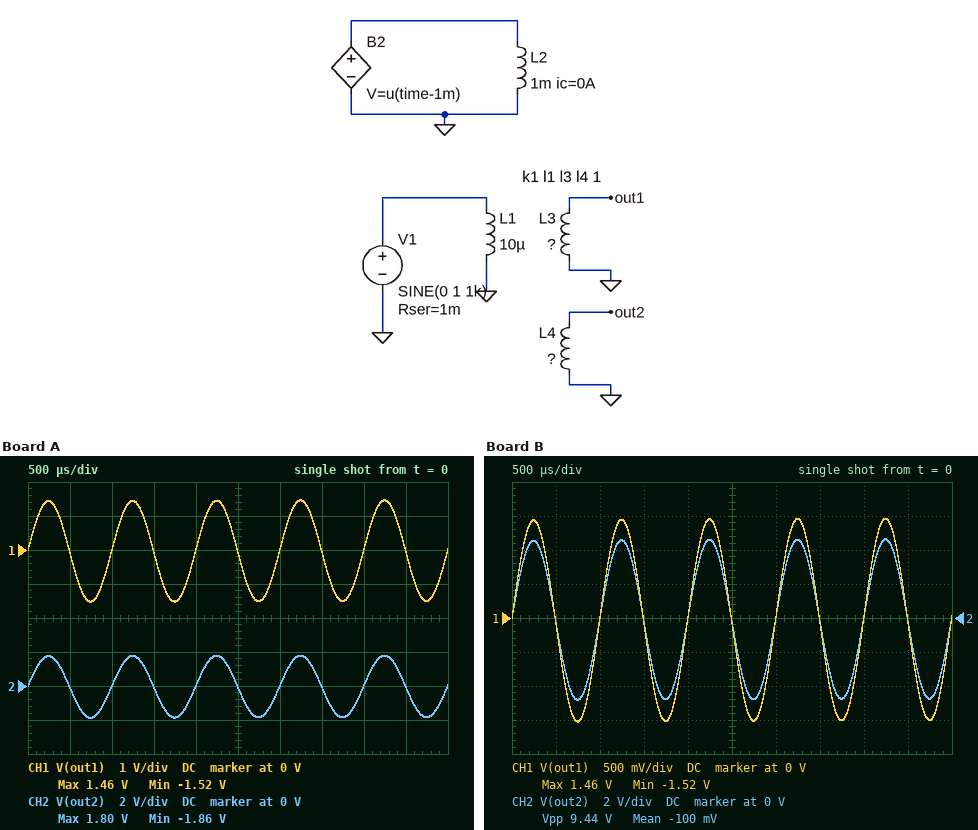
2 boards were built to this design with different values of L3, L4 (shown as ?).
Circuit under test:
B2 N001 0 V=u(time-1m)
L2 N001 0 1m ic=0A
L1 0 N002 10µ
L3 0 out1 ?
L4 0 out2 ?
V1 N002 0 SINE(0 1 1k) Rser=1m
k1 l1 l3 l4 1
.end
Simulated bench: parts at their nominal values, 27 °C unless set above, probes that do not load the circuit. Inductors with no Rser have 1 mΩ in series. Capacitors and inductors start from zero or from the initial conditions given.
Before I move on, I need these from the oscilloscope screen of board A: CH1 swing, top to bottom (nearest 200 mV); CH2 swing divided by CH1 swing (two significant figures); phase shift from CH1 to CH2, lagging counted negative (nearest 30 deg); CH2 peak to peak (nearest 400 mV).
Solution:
3.0 V
1.2
0 deg
3.6 V
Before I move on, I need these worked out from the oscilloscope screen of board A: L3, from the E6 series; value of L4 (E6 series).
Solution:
22 µH
33 µH
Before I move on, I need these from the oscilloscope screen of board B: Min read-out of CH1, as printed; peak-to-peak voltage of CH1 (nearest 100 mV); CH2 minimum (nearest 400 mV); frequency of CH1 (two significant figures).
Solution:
-1.52 V
3.0 V
-4.8 V
1.0 kHz
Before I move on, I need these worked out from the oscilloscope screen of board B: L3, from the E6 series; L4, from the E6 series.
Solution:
22 µH
220 µH
